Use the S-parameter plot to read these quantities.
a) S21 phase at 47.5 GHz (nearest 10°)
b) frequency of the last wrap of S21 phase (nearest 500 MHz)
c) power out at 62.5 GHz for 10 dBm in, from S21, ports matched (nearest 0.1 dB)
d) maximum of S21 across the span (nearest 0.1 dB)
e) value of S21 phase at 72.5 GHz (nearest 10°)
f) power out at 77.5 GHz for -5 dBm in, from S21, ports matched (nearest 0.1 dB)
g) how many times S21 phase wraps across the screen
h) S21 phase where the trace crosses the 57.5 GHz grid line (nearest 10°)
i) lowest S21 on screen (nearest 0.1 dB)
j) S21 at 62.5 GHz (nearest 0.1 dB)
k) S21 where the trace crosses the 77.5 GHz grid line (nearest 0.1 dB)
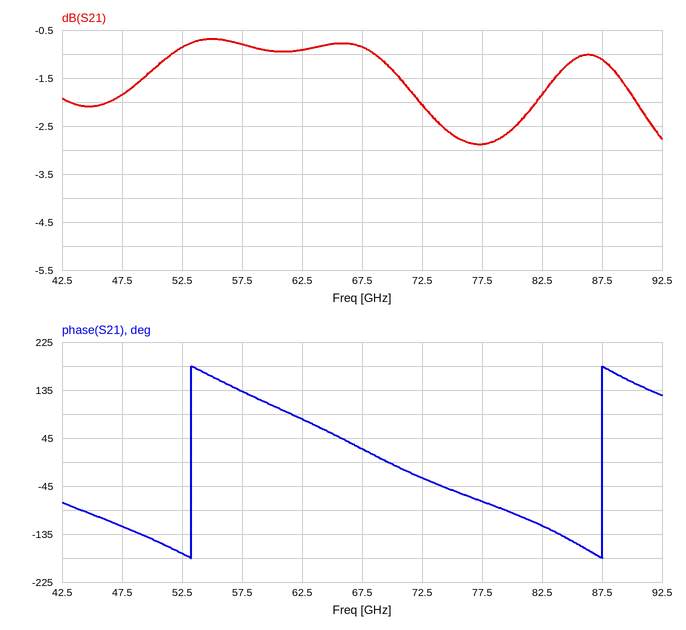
-120°
87.5 GHz
9.1 dBm
-0.7 dB
-30°
-7.9 dBm
2
130°
-2.9 dB
-0.9 dB
-2.9 dB
